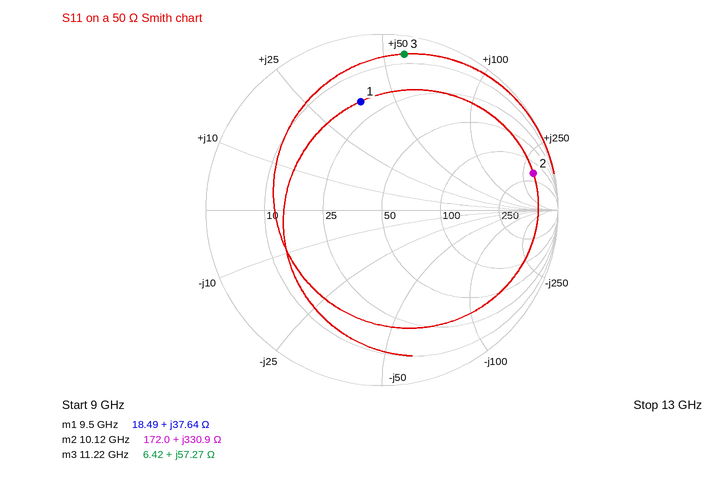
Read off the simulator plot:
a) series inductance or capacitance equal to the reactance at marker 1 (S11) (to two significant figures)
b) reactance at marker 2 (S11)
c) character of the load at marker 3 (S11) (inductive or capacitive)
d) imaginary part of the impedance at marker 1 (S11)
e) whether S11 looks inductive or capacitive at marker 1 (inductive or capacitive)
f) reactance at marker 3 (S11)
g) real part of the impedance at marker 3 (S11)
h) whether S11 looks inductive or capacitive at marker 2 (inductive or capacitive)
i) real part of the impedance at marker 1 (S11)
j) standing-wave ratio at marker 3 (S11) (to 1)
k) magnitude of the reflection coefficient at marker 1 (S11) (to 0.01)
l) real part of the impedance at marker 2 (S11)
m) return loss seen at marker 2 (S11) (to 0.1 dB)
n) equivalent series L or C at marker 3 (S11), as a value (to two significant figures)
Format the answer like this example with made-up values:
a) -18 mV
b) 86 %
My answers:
a) 630 pH
b) +330.9 Ω
c) inductive
d) +37.64 Ω
e) inductive
f) +57.27 Ω
g) 6.42 Ω
h) inductive
i) 18.49 Ω
j) 18
k) 0.63
l) 172.0 Ω
m) 1.1 dB
n) 810 pH
